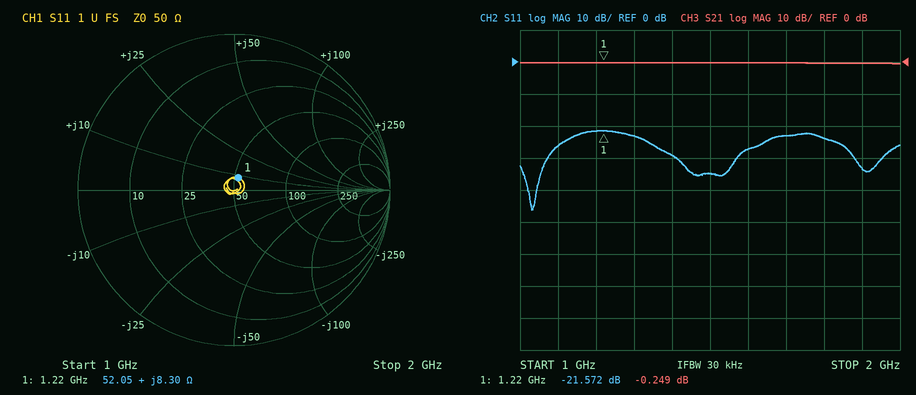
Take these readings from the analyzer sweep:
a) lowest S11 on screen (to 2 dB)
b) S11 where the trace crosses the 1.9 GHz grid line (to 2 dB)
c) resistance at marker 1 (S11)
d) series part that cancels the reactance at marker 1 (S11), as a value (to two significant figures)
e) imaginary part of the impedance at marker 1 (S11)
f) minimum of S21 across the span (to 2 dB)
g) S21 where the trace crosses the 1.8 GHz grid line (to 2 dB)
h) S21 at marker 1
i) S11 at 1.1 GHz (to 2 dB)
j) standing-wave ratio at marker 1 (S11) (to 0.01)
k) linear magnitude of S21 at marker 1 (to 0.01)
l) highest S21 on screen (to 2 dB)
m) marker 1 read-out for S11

-46 dB
-34 dB
52.05 Ω
16 pF
+8.30 Ω
0 dB
0 dB
-0.249 dB
-26 dB
1.18
0.97
0 dB
-21.572 dB
